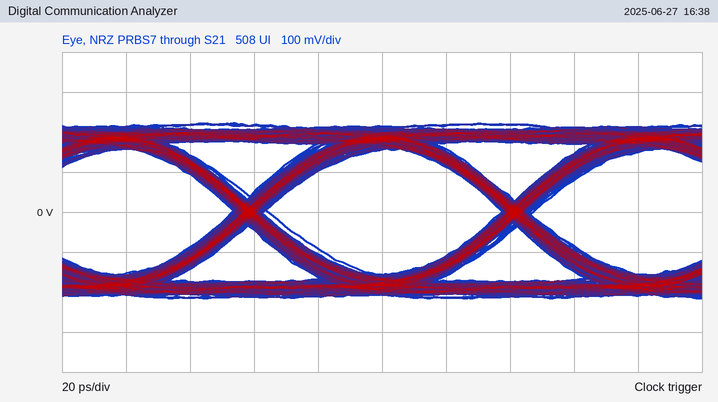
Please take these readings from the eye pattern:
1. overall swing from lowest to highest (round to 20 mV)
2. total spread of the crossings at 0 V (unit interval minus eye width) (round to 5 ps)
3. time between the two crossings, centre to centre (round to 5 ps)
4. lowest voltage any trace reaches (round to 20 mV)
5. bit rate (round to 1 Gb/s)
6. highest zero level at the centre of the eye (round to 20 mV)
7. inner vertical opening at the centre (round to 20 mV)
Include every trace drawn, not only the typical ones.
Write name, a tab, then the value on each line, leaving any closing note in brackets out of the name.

overall swing from lowest to highest	440 mV
total spread of the crossings at 0 V (unit interval minus eye width)	10 ps
time between the two crossings, centre to centre	85 ps
lowest voltage any trace reaches	-220 mV
bit rate	12 Gb/s
highest zero level at the centre of the eye	-160 mV
inner vertical opening at the centre	320 mV
